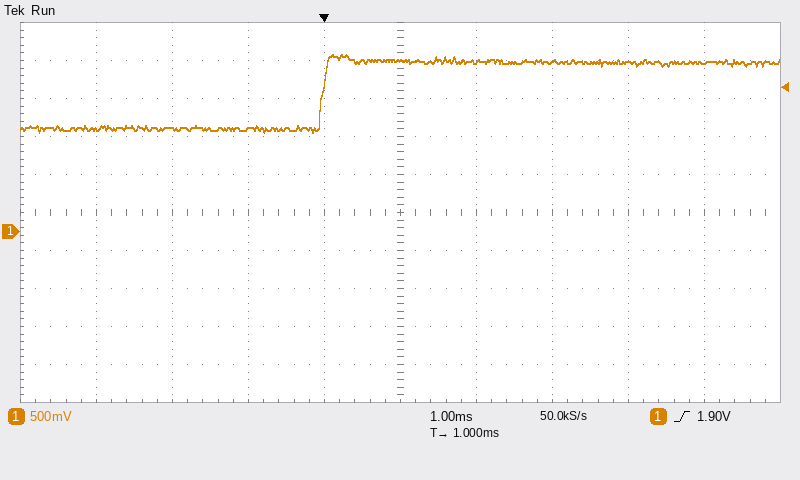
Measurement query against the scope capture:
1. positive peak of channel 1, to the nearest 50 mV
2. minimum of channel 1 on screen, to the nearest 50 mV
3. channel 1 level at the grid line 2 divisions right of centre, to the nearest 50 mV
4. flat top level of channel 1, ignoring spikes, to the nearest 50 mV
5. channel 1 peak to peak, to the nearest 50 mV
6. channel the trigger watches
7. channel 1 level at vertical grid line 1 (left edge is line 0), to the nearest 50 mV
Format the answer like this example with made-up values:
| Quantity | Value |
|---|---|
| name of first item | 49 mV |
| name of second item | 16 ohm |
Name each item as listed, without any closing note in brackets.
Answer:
| Quantity | Value |
|---|---|
| positive peak of channel 1, to the nearest 50 mV | 2.35 V |
| minimum of channel 1 on screen, to the nearest 50 mV | 1.30 V |
| channel 1 level at the grid line 2 divisions right of centre, to the nearest 50 mV | 2.25 V |
| flat top level of channel 1, ignoring spikes, to the nearest 50 mV | 2.25 V |
| channel 1 peak to peak, to the nearest 50 mV | 1.05 V |
| channel the trigger watches | channel 1 |
| channel 1 level at vertical grid line 1 (left edge is line 0), to the nearest 50 mV | 1.35 V |
